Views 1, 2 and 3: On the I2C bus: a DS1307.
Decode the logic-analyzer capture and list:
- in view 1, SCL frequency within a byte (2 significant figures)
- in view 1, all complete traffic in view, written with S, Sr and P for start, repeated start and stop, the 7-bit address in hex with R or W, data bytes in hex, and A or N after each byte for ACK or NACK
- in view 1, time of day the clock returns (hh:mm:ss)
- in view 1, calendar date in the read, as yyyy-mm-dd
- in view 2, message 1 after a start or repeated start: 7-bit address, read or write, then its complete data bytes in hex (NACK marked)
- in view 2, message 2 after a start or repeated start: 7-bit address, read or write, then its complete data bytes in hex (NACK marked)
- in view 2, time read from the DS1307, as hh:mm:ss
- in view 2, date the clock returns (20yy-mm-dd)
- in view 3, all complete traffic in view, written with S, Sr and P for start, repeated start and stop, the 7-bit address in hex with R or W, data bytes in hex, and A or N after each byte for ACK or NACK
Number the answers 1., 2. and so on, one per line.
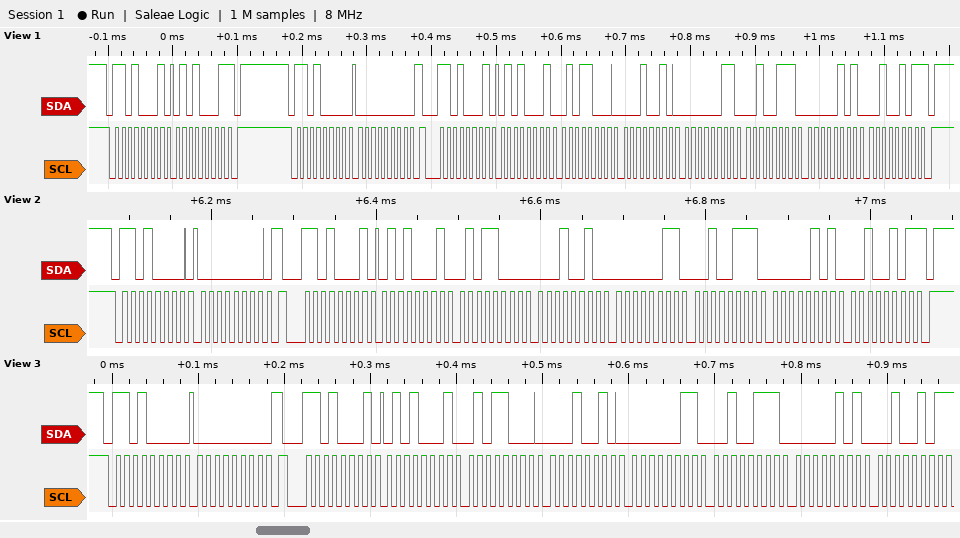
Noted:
1. 100 kHz
2. S 68R A 51 N P S 68W A 00 A Sr 68R A 51 A 58 A 12 A 03 A 27 A 05 A 25 N P
3. 12:58:51
4. 2025-05-27
5. 0x68 write: 00
6. 0x68 read: 51 58 12 03 27 05 25 NACK
7. 12:58:51
8. 2025-05-27
9. S 68W A 00 A Sr 68R A 51 A 58 A 12 A 03 A 27 A 05 A 25 N
